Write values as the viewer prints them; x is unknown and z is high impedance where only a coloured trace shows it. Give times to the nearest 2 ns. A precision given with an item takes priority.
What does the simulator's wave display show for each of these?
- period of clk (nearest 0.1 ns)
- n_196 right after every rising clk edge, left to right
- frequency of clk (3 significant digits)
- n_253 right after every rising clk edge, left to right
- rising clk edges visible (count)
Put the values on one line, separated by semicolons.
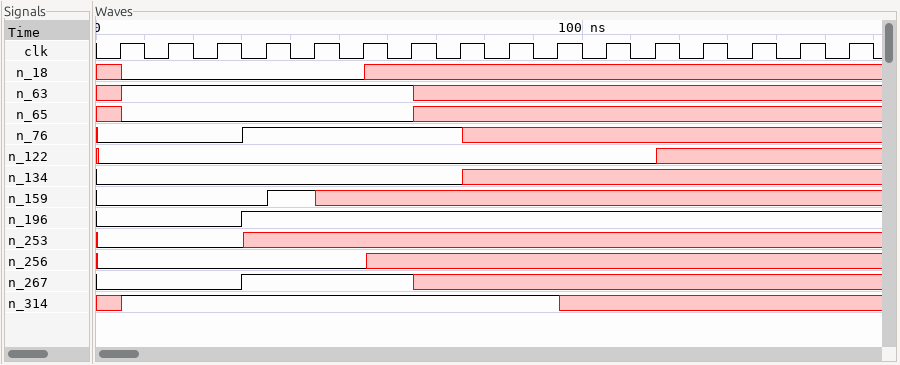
10 ns; 0 0 0 1 1 1 1 1 1 1 1 1 1 1 1 1; 100 MHz; 0 0 0 x x x x x x x x x x x x x; 16
